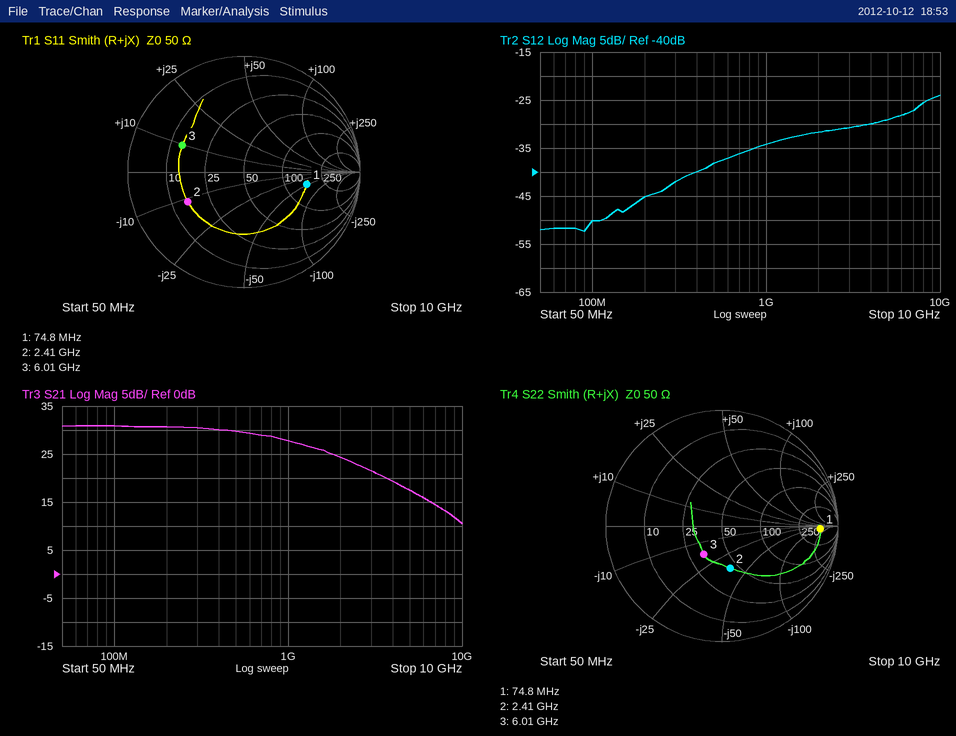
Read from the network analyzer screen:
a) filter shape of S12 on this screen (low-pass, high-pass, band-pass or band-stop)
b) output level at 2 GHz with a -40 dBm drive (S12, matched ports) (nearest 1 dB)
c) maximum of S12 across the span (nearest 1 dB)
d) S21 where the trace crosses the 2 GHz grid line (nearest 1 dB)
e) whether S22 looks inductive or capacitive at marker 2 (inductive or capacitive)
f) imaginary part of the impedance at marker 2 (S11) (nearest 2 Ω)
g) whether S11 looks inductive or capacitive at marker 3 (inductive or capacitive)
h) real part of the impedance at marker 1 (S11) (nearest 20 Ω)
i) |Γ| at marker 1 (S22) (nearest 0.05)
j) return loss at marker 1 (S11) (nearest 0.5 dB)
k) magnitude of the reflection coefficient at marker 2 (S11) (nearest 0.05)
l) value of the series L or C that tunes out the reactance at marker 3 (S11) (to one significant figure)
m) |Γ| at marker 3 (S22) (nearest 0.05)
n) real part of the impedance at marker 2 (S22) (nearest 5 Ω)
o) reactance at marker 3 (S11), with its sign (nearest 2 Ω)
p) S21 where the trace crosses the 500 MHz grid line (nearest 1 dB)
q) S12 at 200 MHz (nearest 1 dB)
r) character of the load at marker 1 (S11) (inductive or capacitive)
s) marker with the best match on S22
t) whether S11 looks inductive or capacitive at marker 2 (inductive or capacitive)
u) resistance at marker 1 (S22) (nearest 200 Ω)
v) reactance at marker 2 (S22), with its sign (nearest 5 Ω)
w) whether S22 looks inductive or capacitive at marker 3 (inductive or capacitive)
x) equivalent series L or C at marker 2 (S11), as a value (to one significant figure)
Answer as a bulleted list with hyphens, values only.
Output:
- high-pass
- -72 dBm
- -24 dB
- 24 dB
- capacitive
- -12 Ω
- inductive
- 160 Ω
- 0.85
- 5.0 dB
- 0.55
- 3 pF
- 0.30
- 45 Ω
- +10 Ω
- 30 dB
- -45 dB
- capacitive
- marker 3
- capacitive
- 600 Ω
- -35 Ω
- capacitive
- 6 pF
